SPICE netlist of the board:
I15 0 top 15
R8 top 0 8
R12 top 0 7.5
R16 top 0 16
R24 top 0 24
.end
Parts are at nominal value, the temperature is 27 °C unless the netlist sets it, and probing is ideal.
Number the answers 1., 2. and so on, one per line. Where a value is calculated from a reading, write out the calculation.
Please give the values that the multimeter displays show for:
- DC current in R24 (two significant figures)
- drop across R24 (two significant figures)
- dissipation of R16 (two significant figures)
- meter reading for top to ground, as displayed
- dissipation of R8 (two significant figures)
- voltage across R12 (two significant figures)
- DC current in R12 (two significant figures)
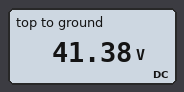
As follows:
1. (41.38 V) / 24 Ω = 1.7 A
2. 41.38 V = 41 V
3. (41.38 V)^2 / 16 Ω = 110 W
4. 41.38 V
5. (41.38 V)^2 / 8 Ω = 210 W
6. 41.38 V = 41 V
7. (41.38 V) / 7.5 Ω = 5.5 A
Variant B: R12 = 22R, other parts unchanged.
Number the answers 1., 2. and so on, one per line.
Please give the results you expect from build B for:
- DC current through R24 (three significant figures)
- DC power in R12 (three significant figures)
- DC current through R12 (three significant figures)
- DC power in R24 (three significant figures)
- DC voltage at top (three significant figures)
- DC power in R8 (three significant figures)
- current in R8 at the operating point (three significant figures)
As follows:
1. 2.28 A
2. 136 W
3. 2.48 A
4. 124 W
5. 54.6 V
6. 373 W
7. 6.83 A
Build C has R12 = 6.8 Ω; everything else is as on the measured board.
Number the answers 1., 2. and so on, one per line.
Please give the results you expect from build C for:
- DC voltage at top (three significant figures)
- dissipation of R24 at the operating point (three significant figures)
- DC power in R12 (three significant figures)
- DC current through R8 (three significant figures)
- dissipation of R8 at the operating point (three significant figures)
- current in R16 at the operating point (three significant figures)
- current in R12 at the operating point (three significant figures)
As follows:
1. 39.9 V
2. 66.2 W
3. 234 W
4. 4.98 A
5. 199 W
6. 2.49 A
7. 5.86 A
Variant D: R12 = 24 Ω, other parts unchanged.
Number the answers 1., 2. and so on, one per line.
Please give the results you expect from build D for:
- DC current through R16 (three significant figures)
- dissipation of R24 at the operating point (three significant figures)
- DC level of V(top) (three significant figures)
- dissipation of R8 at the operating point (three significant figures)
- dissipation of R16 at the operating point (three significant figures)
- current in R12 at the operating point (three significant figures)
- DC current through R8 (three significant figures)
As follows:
1. 3.46 A
2. 128 W
3. 55.4 V
4. 383 W
5. 192 W
6. 2.31 A
7. 6.92 A
